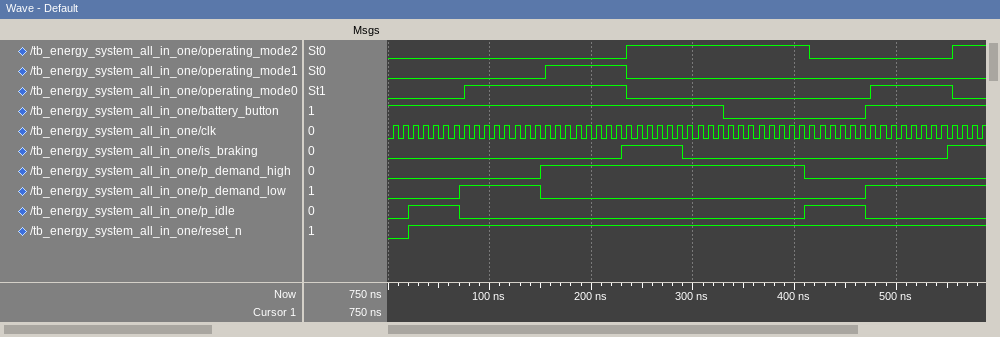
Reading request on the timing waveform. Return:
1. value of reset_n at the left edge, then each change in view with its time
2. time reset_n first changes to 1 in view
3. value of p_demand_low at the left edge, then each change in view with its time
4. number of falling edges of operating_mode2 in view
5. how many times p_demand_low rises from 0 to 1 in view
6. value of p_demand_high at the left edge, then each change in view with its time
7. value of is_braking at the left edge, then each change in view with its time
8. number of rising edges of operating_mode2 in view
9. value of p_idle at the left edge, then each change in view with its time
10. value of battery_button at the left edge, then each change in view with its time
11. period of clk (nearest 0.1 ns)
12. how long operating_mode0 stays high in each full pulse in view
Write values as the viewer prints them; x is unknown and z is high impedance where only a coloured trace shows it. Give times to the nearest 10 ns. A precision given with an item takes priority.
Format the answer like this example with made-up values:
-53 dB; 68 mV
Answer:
0, 1 at 20 ns; 20 ns; 0, 1 at 70 ns, 0 at 150 ns, 1 at 470 ns; 1; 2; 0, 1 at 150 ns, 0 at 410 ns; 0, 1 at 230 ns, 0 at 290 ns, 1 at 550 ns; 2; 0, 1 at 20 ns, 0 at 70 ns, 1 at 410 ns, 0 at 470 ns; 1, 0 at 330 ns, 1 at 470 ns; 10 ns; 160 ns, 80 ns
